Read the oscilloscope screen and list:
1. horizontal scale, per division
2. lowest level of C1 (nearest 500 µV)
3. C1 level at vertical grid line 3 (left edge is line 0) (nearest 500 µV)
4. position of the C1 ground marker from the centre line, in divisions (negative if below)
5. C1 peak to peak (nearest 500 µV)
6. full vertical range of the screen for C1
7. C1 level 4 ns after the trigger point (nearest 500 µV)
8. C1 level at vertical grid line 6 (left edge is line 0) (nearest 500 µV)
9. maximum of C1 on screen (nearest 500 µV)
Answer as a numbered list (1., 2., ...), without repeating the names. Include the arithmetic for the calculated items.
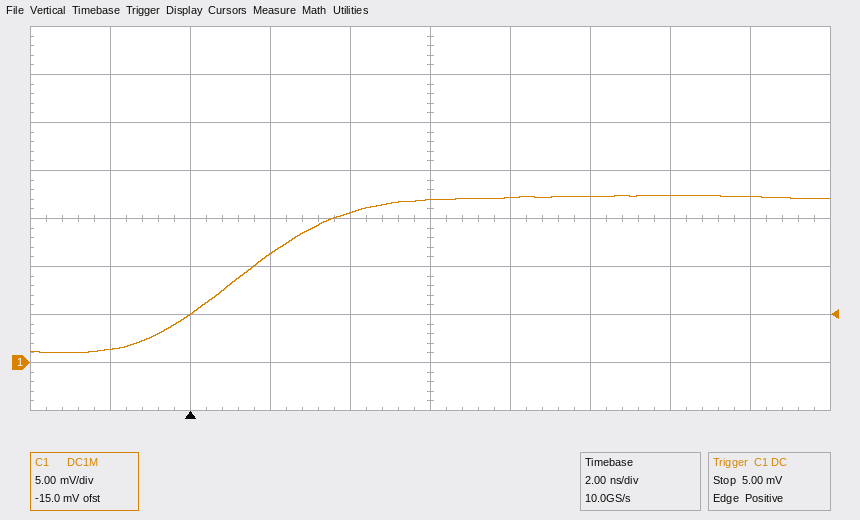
1. 2 ns
2. 1.0 mV
3. 11.5 mV
4. -3.0 div
5. 17.5 mV − (1.0 mV) = 16.5 mV
6. 40 mV
7. 15.5 mV
8. 17.0 mV
9. 17.5 mV
